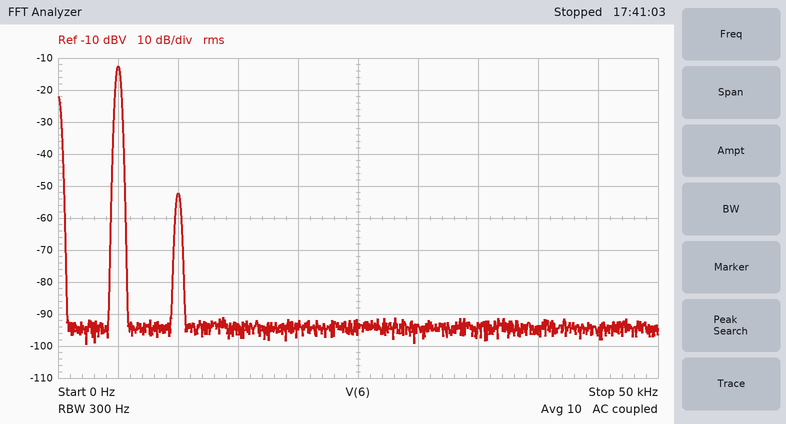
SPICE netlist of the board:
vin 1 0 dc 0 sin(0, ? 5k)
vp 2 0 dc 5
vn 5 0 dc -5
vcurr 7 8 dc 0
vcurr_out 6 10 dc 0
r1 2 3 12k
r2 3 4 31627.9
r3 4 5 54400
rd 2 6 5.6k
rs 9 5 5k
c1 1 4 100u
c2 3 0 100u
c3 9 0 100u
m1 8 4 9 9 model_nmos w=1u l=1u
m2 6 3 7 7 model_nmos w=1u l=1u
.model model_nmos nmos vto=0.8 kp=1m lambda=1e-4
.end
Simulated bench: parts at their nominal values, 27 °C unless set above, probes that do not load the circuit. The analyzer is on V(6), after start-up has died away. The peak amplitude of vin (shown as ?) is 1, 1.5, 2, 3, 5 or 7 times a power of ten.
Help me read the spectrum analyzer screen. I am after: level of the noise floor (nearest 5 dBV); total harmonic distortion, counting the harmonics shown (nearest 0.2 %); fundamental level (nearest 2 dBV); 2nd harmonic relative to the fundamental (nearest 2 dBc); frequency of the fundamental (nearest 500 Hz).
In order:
-95 dBV
1.0 %
-12 dBV
-40 dBc
5.0 kHz
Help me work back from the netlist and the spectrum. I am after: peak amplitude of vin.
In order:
50 mV
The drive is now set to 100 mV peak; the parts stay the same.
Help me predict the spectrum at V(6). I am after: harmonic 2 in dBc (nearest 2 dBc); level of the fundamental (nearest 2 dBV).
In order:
-34 dBc
-6 dBV
